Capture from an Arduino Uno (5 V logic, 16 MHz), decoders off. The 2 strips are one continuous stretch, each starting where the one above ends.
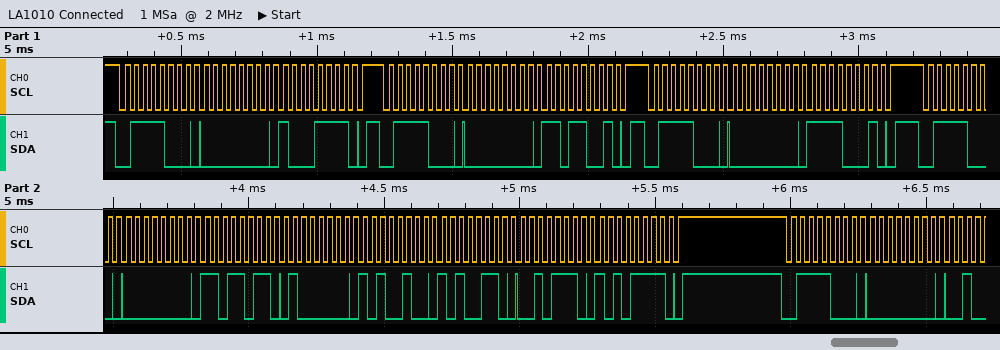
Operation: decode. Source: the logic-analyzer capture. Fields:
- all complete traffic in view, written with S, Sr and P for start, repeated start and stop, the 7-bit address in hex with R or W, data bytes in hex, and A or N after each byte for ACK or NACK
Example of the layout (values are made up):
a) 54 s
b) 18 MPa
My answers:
a) S 3CW A 00 A 8F A P S 3CW A 00 A D9 A P S 3CW A 00 A F1 A P S 3CW A 00 A DB A 40 A A4 A A6 A 2E A AF A P S 3CW A 00 A
